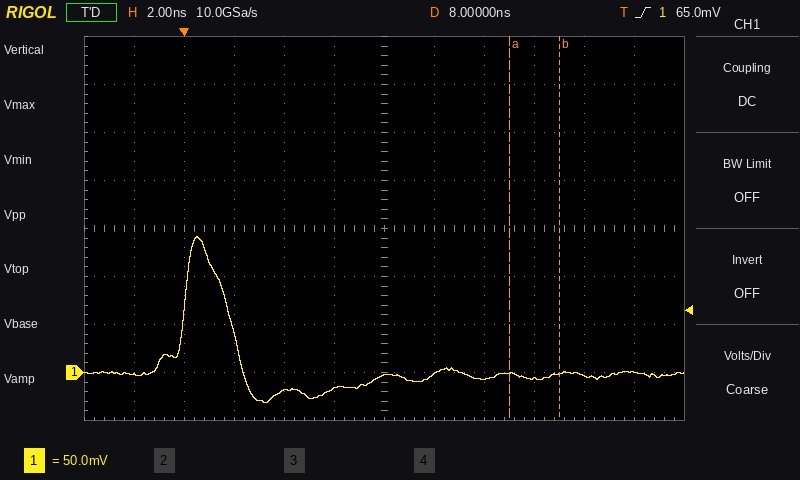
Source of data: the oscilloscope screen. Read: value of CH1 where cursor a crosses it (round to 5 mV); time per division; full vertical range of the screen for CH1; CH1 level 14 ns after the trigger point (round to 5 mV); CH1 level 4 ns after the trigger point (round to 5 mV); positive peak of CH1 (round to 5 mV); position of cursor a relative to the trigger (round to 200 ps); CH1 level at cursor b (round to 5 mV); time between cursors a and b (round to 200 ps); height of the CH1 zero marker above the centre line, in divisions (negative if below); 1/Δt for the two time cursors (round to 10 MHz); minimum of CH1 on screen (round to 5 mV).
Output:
0 mV
2 ns
400 mV
-5 mV
-20 mV
140 mV
+13.0 ns
0 mV
2.0 ns
-3.0 div
500 MHz
-30 mV
